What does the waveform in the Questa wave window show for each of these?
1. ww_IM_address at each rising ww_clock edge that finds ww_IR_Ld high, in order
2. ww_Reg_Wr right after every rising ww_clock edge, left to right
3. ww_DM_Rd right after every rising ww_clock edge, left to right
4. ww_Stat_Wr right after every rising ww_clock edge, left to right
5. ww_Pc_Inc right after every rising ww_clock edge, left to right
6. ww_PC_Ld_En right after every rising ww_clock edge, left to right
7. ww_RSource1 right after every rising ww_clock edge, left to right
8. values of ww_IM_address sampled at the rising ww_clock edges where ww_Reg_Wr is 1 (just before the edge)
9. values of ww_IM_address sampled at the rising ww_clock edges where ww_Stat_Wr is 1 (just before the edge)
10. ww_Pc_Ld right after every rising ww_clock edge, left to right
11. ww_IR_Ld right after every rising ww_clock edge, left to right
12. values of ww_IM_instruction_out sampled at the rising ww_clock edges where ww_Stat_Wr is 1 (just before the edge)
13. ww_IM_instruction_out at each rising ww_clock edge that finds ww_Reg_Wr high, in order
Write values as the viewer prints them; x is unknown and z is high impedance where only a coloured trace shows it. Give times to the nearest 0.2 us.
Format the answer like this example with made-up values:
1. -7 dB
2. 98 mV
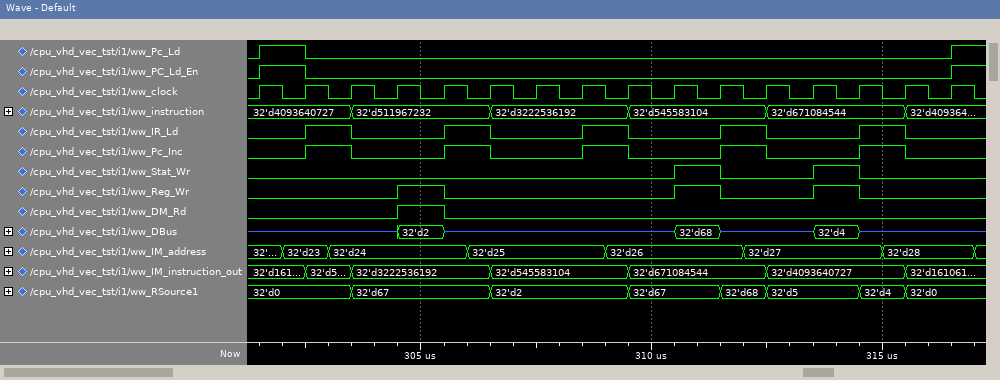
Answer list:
1. 32'd24, 32'd25, 32'd26, 32'd27, 32'd28
2. 0 0 0 1 0 0 0 0 0 1 0 0 1 0 0 0
3. 0 0 0 1 0 0 0 0 0 0 0 0 0 0 0 0
4. 0 0 0 0 0 0 0 0 0 1 0 0 1 0 0 0
5. 0 1 0 0 1 0 0 1 0 0 1 0 0 1 0 0
6. 1 0 0 0 0 0 0 0 0 0 0 0 0 0 0 1
7. 32'd0, 32'd0, 32'd67, 32'd67, 32'd67, 32'd2, 32'd2, 32'd2, 32'd67, 32'd67, 32'd68, 32'd5, 32'd5, 32'd4, 32'd0, 32'd0
8. 32'd24, 32'd26, 32'd27
9. 32'd26, 32'd27
10. 1 0 0 0 0 0 0 0 0 0 0 0 0 0 0 1
11. 0 1 0 0 1 0 0 1 0 0 1 0 0 1 0 0
12. 32'd671084544, 32'd4093640727
13. 32'd3222536192, 32'd671084544, 32'd4093640727
